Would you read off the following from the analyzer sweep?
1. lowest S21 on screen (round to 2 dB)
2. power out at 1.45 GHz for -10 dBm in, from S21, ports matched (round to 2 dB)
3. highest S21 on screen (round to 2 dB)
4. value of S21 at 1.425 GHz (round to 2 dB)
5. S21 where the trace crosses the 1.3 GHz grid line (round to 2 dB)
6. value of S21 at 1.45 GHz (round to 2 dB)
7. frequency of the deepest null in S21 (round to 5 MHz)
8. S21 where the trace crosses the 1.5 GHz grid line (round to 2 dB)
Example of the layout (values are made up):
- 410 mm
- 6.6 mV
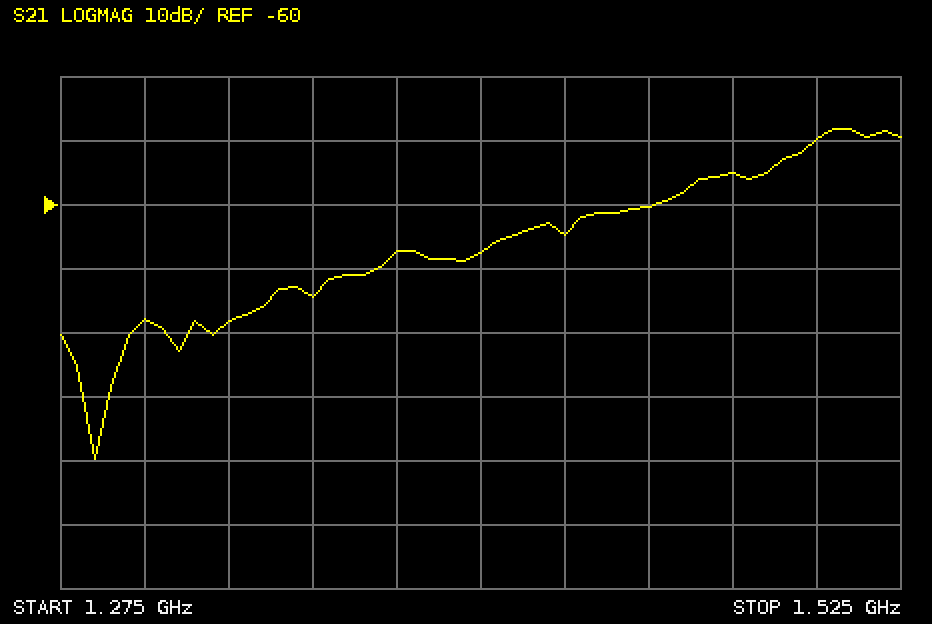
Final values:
- -100 dB
- -70 dBm
- -48 dB
- -64 dB
- -78 dB
- -60 dB
- 1.285 GHz
- -50 dB
